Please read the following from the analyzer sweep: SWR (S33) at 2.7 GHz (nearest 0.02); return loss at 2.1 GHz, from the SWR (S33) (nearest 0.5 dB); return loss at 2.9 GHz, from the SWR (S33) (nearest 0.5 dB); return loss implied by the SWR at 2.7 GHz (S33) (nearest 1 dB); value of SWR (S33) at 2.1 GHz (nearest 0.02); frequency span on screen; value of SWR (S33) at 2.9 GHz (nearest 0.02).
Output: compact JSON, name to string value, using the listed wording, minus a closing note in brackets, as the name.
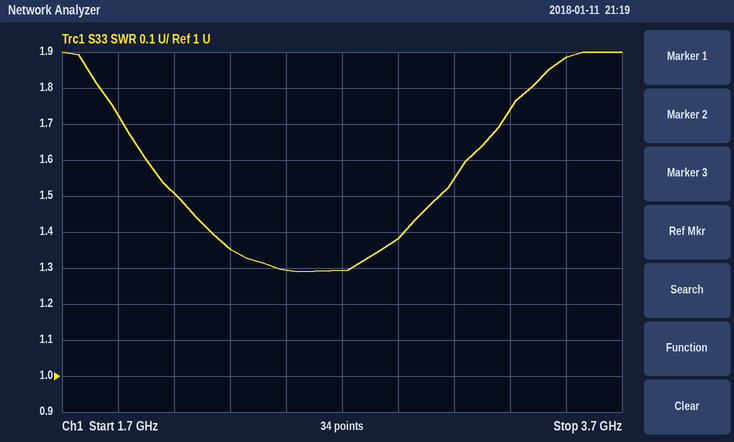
{"SWR (S33) at 2.7 GHz": "1.30", "return loss at 2.1 GHz, from the SWR (S33)": "14.0 dB", "return loss at 2.9 GHz, from the SWR (S33)": "16.0 dB", "return loss implied by the SWR at 2.7 GHz (S33)": "18 dB", "value of SWR (S33) at 2.1 GHz": "1.50", "frequency span on screen": "2 GHz", "value of SWR (S33) at 2.9 GHz": "1.38"}
